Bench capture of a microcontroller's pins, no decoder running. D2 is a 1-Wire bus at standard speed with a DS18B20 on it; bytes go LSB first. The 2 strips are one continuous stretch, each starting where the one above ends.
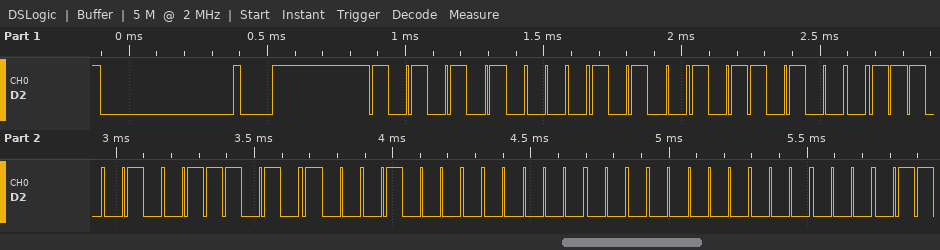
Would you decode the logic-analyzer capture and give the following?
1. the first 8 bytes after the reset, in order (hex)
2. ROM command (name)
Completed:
55 28 2D 4E AE 08 00 00
Match ROM
